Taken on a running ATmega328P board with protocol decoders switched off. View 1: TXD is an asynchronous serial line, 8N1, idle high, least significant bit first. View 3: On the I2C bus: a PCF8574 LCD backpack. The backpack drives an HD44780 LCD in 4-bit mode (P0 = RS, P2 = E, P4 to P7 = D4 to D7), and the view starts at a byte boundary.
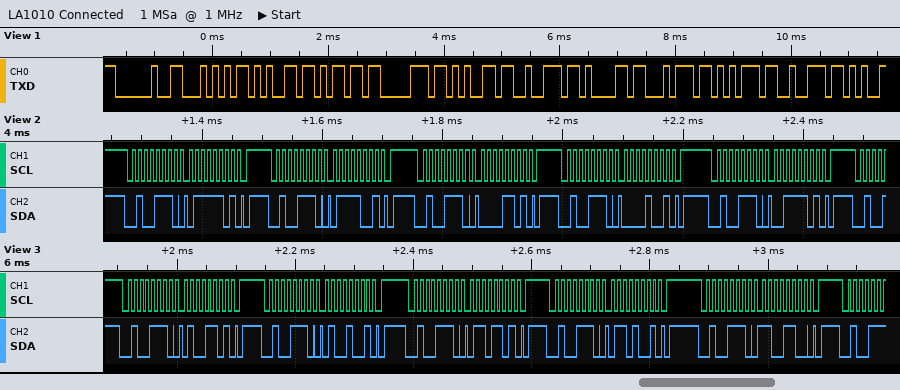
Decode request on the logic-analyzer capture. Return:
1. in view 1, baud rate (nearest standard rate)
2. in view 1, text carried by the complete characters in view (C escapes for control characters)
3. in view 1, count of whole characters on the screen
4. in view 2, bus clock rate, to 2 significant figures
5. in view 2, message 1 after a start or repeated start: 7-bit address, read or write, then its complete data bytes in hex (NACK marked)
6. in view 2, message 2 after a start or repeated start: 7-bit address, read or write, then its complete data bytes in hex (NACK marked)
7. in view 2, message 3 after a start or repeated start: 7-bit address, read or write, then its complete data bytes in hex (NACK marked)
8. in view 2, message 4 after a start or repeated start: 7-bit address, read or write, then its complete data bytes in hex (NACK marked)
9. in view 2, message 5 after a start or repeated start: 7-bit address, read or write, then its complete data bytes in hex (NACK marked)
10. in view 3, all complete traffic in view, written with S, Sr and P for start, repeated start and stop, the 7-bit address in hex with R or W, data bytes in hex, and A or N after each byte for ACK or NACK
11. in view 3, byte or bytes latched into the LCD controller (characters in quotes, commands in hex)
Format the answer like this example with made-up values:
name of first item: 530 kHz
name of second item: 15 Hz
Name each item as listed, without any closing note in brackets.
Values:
in view 1, baud rate: 9600 baud
in view 1, text carried by the complete characters in view: " Temperatur"
in view 1, count of whole characters on the screen: 11
in view 2, bus clock rate, to 2 significant figures: 100 kHz
in view 2, message 1 after a start or repeated start: 7-bit address, read or write, then its complete data bytes in hex: 0x27 write: 7D
in view 2, message 2 after a start or repeated start: 7-bit address, read or write, then its complete data bytes in hex: 0x27 write: 79
in view 2, message 3 after a start or repeated start: 7-bit address, read or write, then its complete data bytes in hex: 0x27 write: 0D
in view 2, message 4 after a start or repeated start: 7-bit address, read or write, then its complete data bytes in hex: 0x27 write: 09
in view 2, message 5 after a start or repeated start: 7-bit address, read or write, then its complete data bytes in hex: 0x27 write: 3D
in view 3, all complete traffic in view, written with S, Sr and P for start, repeated start and stop, the 7-bit address in hex with R or W, data bytes in hex, and A or N after each byte for ACK or NACK: S 27W A 4D A P S 27W A 49 A P S 27W A 6D A P S 27W A 69 A P S 27W A CC A P
in view 3, byte or bytes latched into the LCD controller: 'F'
